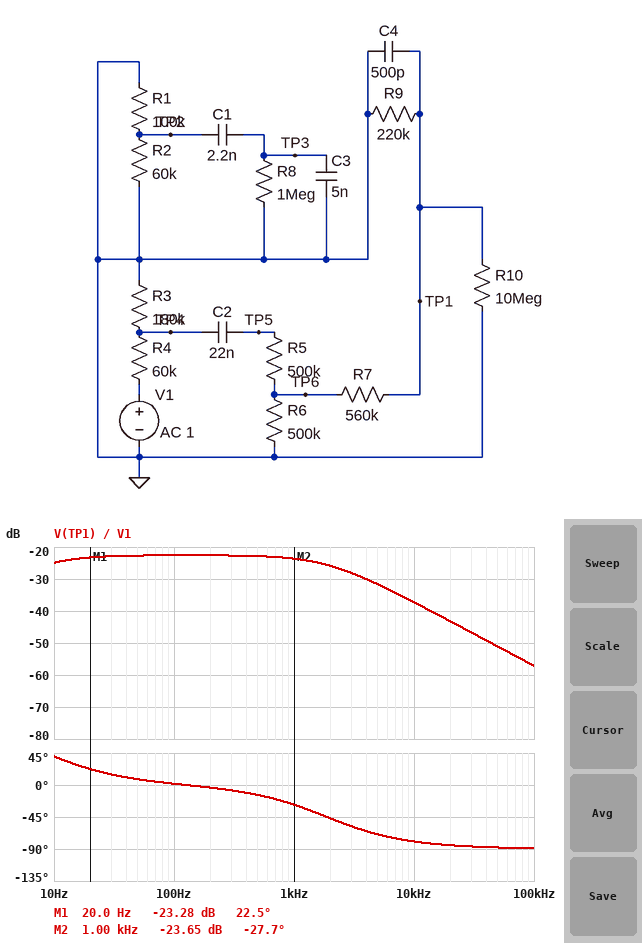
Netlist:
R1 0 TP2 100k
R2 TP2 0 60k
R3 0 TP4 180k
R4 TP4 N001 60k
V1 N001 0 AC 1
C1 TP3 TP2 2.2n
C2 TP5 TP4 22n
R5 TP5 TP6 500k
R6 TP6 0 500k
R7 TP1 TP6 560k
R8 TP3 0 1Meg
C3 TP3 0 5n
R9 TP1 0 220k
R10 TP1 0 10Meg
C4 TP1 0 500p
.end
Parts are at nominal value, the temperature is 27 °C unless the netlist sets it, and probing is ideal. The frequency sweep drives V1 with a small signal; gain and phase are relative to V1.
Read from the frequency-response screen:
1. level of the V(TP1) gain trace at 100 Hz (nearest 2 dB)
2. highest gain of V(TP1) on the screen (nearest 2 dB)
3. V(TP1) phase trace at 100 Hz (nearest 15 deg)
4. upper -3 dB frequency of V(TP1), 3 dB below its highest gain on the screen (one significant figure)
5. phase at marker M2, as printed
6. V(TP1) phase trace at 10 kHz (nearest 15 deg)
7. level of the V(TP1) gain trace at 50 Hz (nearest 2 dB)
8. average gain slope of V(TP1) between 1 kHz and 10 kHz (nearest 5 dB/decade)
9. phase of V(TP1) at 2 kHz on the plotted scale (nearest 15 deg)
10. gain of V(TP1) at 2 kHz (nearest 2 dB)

-22 dB
-22 dB
0 deg
2 kHz
-27.7 deg
-75 deg
-22 dB
-15 dB/decade
-45 deg
-26 dB
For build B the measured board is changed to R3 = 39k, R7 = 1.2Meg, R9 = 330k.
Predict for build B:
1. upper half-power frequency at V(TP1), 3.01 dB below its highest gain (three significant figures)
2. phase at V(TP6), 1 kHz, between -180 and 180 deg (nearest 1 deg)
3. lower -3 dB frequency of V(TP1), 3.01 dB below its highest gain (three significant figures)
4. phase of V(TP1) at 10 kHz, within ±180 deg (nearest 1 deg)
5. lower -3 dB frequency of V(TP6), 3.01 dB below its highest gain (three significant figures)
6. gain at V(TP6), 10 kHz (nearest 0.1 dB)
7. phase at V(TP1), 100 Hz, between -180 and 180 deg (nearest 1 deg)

1.23 kHz
-1 deg
7.93 Hz
-83 deg
8.01 Hz
-16.0 dB
0 deg
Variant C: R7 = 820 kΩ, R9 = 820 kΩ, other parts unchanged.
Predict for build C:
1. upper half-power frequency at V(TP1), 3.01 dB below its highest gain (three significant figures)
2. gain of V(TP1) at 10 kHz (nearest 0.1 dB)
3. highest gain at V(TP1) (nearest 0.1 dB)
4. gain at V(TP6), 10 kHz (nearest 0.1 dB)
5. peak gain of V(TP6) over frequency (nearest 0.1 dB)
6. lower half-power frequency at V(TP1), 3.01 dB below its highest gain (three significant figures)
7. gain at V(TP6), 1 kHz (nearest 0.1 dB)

731 Hz
-39.5 dB
-16.7 dB
-11.3 dB
-10.3 dB
7.65 Hz
-10.9 dB
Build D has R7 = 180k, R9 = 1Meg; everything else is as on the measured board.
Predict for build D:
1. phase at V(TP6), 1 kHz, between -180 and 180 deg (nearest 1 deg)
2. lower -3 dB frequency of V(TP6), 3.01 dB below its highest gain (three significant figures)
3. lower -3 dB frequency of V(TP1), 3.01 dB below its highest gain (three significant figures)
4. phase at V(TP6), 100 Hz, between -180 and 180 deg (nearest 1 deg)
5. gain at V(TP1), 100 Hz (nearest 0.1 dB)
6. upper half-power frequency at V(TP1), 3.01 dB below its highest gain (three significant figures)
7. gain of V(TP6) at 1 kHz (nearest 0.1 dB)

-17 deg
8.03 Hz
8.01 Hz
2 deg
-12.4 dB
1.09 kHz
-12.6 dB
